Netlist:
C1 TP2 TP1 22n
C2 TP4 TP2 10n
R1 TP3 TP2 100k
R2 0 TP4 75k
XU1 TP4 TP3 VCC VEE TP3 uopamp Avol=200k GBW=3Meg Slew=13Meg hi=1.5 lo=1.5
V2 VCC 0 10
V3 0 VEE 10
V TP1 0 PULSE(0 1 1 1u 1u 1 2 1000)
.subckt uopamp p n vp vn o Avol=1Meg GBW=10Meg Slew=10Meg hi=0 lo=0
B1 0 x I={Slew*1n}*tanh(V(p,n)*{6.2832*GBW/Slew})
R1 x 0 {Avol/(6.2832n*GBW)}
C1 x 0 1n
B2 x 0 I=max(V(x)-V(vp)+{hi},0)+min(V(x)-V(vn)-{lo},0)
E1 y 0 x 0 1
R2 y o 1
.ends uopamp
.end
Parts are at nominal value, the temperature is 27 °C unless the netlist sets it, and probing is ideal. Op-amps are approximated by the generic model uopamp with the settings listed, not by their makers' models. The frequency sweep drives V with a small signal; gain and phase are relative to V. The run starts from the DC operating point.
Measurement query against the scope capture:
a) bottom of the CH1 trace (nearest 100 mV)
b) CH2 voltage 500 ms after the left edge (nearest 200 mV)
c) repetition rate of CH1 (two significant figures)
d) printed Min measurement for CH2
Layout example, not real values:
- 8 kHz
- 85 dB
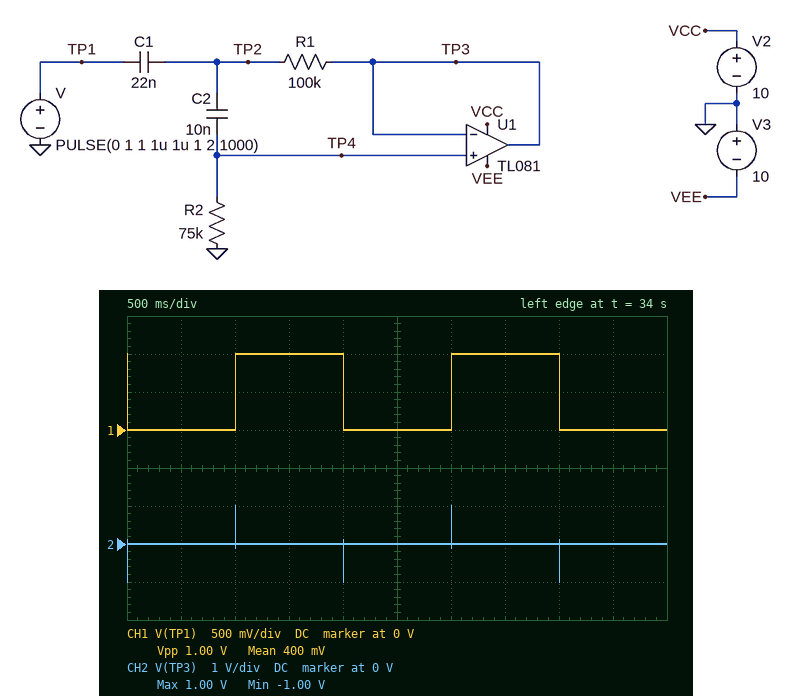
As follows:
- 0 V
- 0 V
- 500 mHz
- -1.00 V
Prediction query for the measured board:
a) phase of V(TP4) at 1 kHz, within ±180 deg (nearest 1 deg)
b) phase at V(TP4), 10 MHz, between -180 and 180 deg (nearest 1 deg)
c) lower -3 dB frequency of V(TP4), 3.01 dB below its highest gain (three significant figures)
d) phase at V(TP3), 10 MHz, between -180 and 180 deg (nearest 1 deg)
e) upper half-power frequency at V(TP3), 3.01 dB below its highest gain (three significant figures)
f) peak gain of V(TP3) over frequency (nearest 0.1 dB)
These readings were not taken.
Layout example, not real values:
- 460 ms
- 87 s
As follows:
- 17 deg
- 0 deg
- 261 Hz
- -73 deg
- 3.00 MHz
- 0 dB
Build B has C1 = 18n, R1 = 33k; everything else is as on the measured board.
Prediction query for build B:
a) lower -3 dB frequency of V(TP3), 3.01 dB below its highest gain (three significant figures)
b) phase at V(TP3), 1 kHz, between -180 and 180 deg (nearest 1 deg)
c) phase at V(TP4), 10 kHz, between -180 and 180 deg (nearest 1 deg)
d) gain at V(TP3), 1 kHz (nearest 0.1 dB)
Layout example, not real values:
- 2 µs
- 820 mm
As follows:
- 234 Hz
- 19 deg
- 2 deg
- 0 dB
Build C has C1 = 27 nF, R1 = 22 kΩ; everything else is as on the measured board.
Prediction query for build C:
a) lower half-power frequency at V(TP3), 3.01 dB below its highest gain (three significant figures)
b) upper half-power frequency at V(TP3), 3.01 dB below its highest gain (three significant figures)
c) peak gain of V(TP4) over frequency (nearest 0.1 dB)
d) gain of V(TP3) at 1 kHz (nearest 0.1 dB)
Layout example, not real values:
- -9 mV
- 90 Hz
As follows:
- 216 Hz
- 2.80 MHz
- 0.3 dB
- 0.1 dB
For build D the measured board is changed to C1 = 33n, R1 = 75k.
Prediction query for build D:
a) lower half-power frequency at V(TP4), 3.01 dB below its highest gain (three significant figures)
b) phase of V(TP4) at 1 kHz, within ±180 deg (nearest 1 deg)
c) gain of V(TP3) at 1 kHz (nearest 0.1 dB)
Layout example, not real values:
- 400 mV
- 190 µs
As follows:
- 230 Hz
- 16 deg
- -0.2 dB
